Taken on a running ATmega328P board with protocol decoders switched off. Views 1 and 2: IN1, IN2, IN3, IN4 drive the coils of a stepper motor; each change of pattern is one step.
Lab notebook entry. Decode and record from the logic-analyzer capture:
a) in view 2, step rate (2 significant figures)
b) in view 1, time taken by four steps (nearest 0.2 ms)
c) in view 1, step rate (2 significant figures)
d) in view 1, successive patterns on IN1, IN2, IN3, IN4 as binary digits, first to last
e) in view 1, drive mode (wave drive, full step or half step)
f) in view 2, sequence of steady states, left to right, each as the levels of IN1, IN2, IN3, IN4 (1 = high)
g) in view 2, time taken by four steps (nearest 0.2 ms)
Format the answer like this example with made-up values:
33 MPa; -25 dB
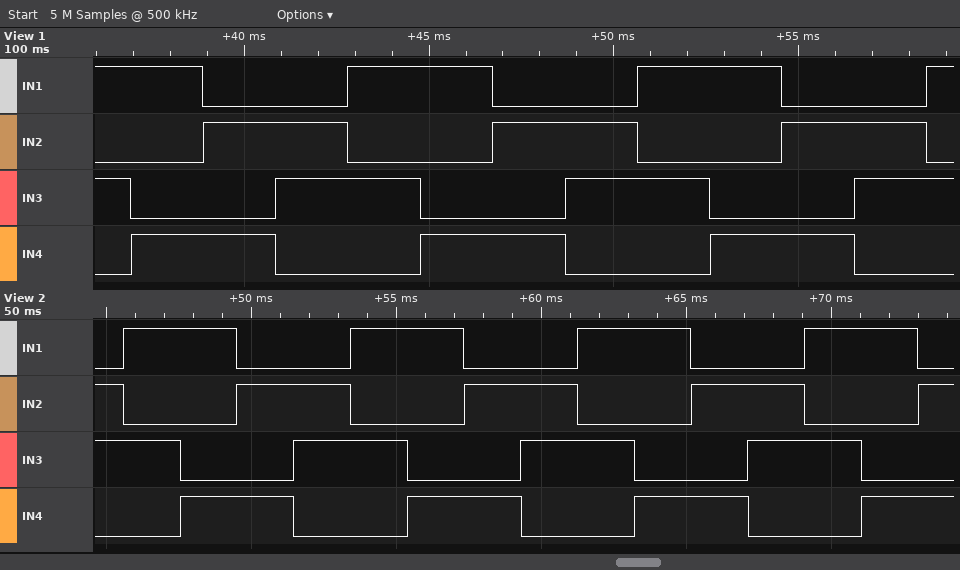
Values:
510 steps/s; 7.8 ms; 510 steps/s; 1010 1001 0101 0110 1010 1001 0101 0110 1010 1001 0101 0110 1010; full step; 0110 1010 1001 0101 0110 1010 1001 0101 0110 1010 1001 0101 0110 1010 1001 0101; 7.8 ms
